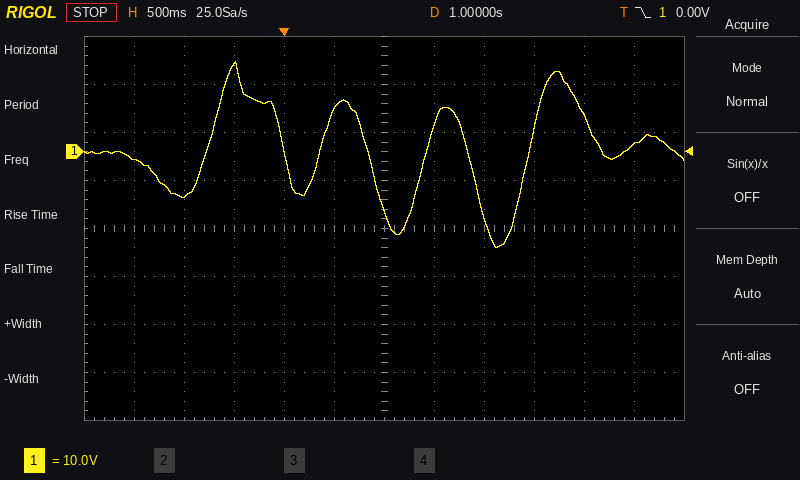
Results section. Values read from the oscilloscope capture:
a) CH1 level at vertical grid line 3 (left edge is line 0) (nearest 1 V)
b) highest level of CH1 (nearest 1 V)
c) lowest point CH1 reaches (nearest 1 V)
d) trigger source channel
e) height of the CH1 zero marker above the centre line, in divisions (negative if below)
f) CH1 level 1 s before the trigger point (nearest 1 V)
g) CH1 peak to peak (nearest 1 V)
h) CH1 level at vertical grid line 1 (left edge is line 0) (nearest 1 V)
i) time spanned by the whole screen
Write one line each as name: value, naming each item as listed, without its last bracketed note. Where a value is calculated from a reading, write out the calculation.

CH1 level at vertical grid line 3 (left edge is line 0): 18 V
highest level of CH1: 19 V
lowest point CH1 reaches: -20 V
trigger source channel: CH1
height of the CH1 zero marker above the centre line, in divisions: +1.6 div
CH1 level 1 s before the trigger point: -9 V
CH1 peak to peak: 19 V − (-20 V) = 39 V
CH1 level at vertical grid line 1 (left edge is line 0): -2 V
time spanned by the whole screen: 6 s
